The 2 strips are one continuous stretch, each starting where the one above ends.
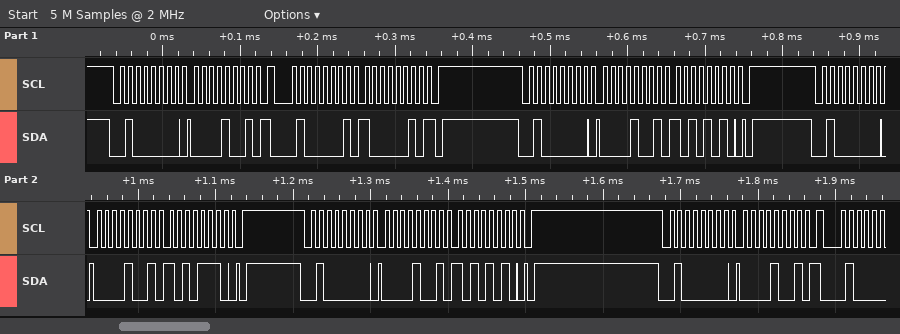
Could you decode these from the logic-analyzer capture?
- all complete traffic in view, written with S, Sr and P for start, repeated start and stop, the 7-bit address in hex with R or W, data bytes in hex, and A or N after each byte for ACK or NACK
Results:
S 20W A 09 A Sr 20R A 82 N P S 20W A 09 A AA A P S 20W A 09 A AE A P S 20W A 09 A AA A P S 20W A 09 A
